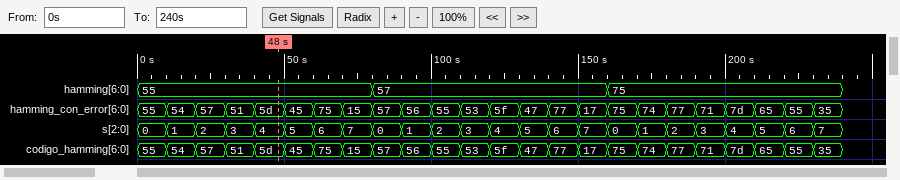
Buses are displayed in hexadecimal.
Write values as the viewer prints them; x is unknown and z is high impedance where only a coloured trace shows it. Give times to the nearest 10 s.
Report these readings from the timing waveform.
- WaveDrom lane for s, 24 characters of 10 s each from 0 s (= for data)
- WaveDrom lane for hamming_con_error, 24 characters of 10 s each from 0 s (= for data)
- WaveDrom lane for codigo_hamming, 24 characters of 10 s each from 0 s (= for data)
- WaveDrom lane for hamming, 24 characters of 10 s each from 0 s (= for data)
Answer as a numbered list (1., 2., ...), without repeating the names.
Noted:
1. {name: 's', wave: '========================', data: '0 1 2 3 4 5 6 7 0 1 2 3 4 5 6 7 0 1 2 3 4 5 6 7'}
2. {name: 'hamming_con_error', wave: '========================', data: '55 54 57 51 5d 45 75 15 57 56 55 53 5f 47 77 17 75 74 77 71 7d 65 55 35'}
3. {name: 'codigo_hamming', wave: '========================', data: '55 54 57 51 5d 45 75 15 57 56 55 53 5f 47 77 17 75 74 77 71 7d 65 55 35'}
4. {name: 'hamming', wave: '=.......=.......=.......', data: '55 57 75'}
